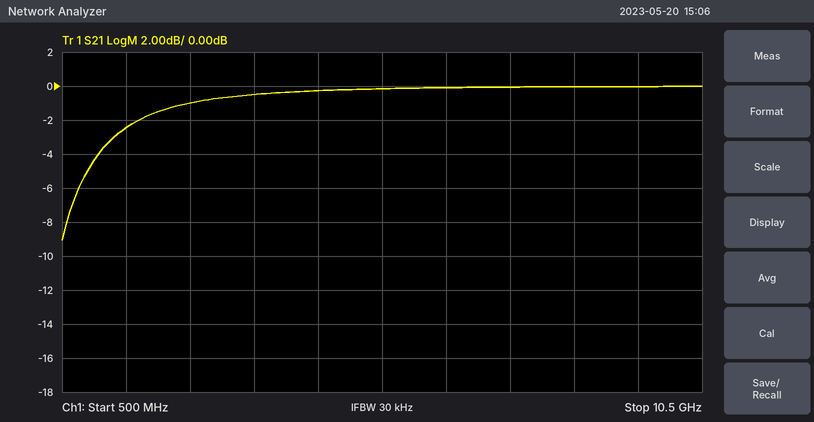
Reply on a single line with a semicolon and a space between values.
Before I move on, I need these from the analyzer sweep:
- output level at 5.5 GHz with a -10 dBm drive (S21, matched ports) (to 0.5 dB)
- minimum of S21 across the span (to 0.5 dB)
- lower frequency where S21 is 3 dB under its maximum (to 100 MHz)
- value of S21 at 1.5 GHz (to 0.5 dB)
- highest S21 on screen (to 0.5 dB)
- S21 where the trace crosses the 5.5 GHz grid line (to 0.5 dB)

-10.0 dBm; -9.0 dB; 1.3 GHz; -2.5 dB; 0.0 dB; 0.0 dB
